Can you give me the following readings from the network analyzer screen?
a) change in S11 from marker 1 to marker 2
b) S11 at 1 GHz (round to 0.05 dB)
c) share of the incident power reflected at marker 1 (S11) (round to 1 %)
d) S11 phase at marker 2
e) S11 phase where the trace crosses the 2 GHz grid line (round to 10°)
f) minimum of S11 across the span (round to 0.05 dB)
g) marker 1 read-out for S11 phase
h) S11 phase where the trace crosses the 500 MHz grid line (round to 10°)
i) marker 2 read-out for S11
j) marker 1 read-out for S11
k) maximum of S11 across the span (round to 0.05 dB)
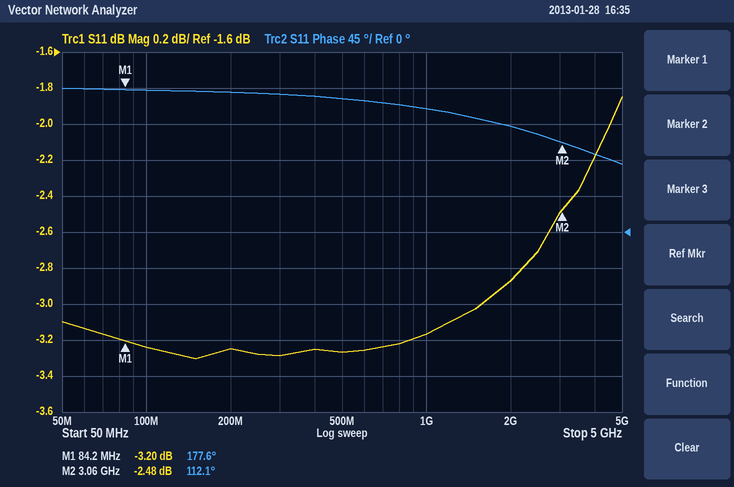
0.72 dB
-3.15 dB
48 %
112.1°
130°
-3.30 dB
177.6°
170°
-2.48 dB
-3.20 dB
-1.85 dB
